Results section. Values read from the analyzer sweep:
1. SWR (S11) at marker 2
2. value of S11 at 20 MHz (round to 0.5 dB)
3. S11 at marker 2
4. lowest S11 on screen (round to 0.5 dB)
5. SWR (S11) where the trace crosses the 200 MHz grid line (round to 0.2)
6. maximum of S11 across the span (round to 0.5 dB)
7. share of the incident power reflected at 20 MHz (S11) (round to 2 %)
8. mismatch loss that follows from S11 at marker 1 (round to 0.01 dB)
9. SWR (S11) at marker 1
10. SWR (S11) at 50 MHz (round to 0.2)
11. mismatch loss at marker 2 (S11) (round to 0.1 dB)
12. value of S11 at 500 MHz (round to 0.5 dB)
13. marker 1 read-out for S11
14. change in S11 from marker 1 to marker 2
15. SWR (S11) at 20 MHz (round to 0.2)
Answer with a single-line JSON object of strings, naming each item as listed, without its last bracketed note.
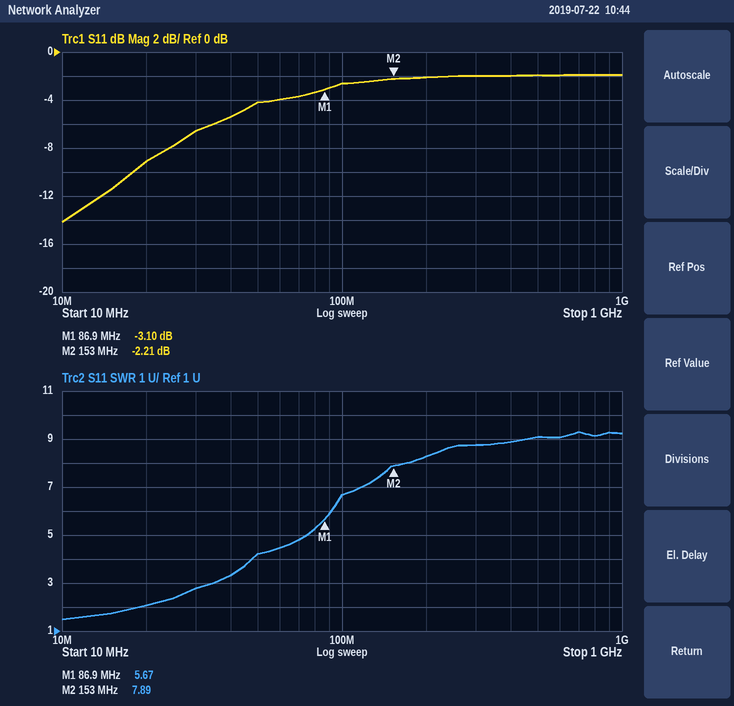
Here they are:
{"SWR (S11) at marker 2": "7.89", "value of S11 at 20 MHz": "-9.0 dB", "S11 at marker 2": "-2.21 dB", "lowest S11 on screen": "-14.0 dB", "SWR (S11) where the trace crosses the 200 MHz grid line": "8.2", "maximum of S11 across the span": "-2.0 dB", "share of the incident power reflected at 20 MHz (S11)": "12 %", "mismatch loss that follows from S11 at marker 1": "2.92 dB", "SWR (S11) at marker 1": "5.67", "SWR (S11) at 50 MHz": "4.2", "mismatch loss at marker 2 (S11)": "4.0 dB", "value of S11 at 500 MHz": "-2.0 dB", "marker 1 read-out for S11": "-3.10 dB", "change in S11 from marker 1 to marker 2": "0.89 dB", "SWR (S11) at 20 MHz": "2.0"}
